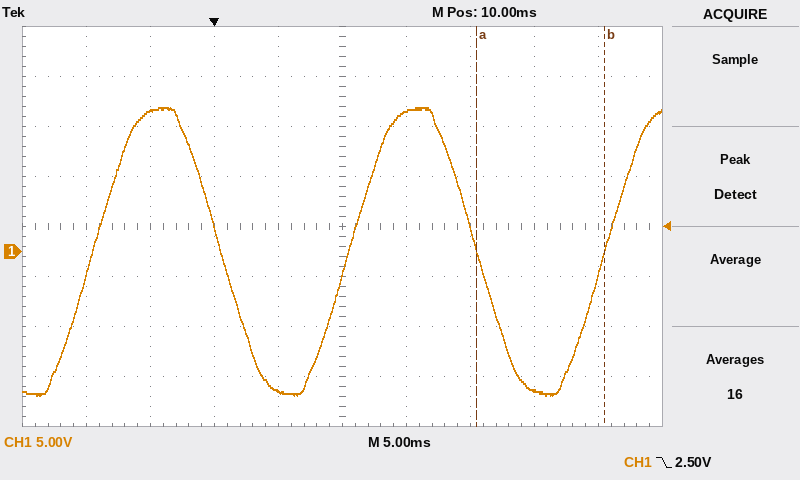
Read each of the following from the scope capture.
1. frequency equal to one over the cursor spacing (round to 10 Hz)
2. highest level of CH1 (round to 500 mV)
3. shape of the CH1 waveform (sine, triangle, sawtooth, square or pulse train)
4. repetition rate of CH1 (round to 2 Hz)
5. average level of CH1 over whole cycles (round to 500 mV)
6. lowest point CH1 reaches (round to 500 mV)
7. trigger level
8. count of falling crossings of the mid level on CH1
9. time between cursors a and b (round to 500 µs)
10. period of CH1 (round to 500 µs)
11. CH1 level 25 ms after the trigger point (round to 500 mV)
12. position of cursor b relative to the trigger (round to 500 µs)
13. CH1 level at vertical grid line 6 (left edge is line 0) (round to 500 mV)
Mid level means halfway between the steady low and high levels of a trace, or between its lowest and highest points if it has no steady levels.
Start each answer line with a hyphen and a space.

- 100 Hz
- 14.5 V
- sine
- 50 Hz
- 0.0 V
- -14.5 V
- 2.50 V
- 2
- 10.0 ms
- 20.0 ms
- -14.0 V
- +30.5 ms
- 14.0 V
